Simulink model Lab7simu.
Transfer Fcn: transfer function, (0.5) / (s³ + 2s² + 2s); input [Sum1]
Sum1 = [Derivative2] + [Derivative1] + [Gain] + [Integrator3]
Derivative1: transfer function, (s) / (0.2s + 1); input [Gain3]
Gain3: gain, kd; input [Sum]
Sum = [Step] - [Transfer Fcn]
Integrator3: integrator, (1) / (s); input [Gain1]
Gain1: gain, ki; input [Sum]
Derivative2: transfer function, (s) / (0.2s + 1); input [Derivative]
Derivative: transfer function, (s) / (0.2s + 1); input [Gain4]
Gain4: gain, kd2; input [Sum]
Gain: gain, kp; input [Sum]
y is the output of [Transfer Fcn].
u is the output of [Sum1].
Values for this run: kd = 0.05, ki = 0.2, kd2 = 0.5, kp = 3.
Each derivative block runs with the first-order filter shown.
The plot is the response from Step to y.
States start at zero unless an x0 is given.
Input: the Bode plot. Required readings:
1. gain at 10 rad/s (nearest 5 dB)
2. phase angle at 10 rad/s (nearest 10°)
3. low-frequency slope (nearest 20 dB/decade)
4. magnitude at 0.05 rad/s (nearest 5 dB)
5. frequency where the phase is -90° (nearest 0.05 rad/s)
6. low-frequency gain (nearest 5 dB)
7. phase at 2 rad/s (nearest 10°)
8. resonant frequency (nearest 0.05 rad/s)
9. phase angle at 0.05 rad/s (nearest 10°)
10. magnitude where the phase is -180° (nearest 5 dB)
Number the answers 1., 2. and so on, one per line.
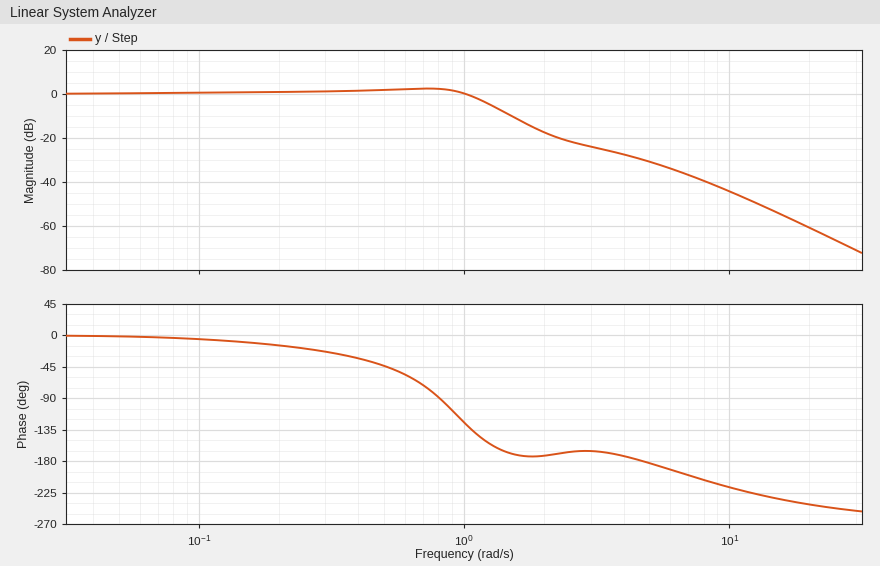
1. -45 dB
2. -220°
3. 0 dB/decade
4. 0 dB
5. 0.80 rad/s
6. 0 dB
7. -170°
8. 0.70 rad/s
9. 0°
10. -30 dB
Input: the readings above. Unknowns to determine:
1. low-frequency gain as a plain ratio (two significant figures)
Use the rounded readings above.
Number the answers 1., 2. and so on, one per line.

1. 1.0
